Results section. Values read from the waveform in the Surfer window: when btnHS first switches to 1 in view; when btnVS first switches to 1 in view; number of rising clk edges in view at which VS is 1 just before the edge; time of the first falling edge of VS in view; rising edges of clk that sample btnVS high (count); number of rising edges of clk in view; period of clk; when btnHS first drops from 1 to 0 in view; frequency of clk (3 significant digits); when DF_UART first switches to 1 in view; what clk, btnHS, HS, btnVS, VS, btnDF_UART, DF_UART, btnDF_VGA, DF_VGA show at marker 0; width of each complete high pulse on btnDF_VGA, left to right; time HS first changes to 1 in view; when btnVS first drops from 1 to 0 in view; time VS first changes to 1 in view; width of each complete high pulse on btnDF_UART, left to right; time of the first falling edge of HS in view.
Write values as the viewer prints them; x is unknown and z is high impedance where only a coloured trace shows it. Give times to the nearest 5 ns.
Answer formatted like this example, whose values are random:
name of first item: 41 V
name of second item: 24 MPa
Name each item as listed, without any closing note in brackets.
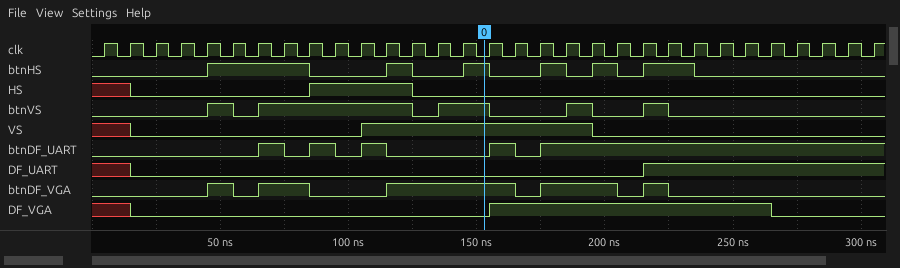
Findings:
when btnHS first switches to 1 in view: 45 ns
when btnVS first switches to 1 in view: 45 ns
number of rising clk edges in view at which VS is 1 just before the edge: 9
time of the first falling edge of VS in view: 195 ns
rising edges of clk that sample btnVS high: 11
number of rising edges of clk in view: 31
period of clk: 10 ns
when btnHS first drops from 1 to 0 in view: 85 ns
frequency of clk: 100 MHz
when DF_UART first switches to 1 in view: 215 ns
what clk, btnHS, HS, btnVS, VS, btnDF_UART, DF_UART, btnDF_VGA, DF_VGA show at marker 0: clk=0, btnHS=1, HS=0, btnVS=1, VS=1, btnDF_UART=0, DF_UART=0, btnDF_VGA=1, DF_VGA=0
width of each complete high pulse on btnDF_VGA, left to right: 10 ns, 20 ns, 50 ns, 30 ns, 10 ns
time HS first changes to 1 in view: 85 ns
when btnVS first drops from 1 to 0 in view: 55 ns
time VS first changes to 1 in view: 105 ns
width of each complete high pulse on btnDF_UART, left to right: 10 ns, 10 ns, 10 ns, 10 ns
time of the first falling edge of HS in view: 125 ns
